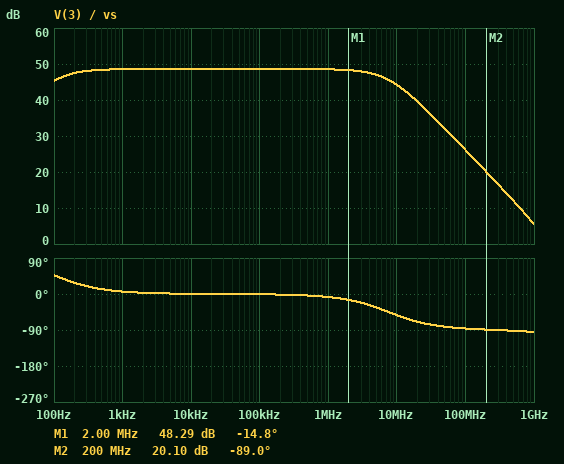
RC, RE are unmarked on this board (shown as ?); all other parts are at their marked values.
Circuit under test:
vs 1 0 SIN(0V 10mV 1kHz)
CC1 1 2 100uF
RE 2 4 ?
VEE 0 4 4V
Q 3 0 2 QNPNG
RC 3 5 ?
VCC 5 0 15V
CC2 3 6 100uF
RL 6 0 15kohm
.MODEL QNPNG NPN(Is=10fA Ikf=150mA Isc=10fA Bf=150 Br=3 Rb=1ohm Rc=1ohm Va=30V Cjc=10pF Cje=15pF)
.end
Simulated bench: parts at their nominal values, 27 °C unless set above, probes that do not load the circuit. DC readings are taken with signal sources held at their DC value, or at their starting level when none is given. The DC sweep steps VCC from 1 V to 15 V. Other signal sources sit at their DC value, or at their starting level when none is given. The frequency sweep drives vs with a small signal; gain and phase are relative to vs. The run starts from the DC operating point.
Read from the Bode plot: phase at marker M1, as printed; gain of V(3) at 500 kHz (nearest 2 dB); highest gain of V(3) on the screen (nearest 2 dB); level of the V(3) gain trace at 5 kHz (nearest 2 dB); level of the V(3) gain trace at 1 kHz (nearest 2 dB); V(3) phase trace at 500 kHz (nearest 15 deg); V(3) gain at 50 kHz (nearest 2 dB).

-14.8 deg
48 dB
48 dB
48 dB
48 dB
0 deg
48 dB
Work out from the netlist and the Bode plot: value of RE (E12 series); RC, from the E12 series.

1.5 kΩ
5.6 kΩ
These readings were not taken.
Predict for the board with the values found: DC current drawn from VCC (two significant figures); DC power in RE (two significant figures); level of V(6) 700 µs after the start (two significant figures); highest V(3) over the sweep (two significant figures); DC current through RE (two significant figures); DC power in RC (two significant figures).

2.2 mA
7.4 mW
-3.0 V
2.7 V
2.2 mA
27 mW
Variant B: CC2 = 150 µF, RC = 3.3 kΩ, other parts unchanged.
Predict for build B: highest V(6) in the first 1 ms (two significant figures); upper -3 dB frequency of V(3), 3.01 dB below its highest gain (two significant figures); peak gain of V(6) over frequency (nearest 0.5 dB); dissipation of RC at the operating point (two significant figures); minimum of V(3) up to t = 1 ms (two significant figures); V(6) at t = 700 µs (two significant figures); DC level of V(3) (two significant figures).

1.6 V
14 MHz
46.0 dB
16 mW
5.4 V
-2.3 V
7.7 V
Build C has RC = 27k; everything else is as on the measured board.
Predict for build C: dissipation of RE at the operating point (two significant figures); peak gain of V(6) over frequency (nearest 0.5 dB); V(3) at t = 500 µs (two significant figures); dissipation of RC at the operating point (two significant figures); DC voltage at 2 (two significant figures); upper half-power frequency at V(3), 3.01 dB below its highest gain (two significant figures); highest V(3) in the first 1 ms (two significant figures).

7.2 mW
0.5 dB
-700 mV
9.1 mW
-710 mV
1.5 GHz
-690 mV
